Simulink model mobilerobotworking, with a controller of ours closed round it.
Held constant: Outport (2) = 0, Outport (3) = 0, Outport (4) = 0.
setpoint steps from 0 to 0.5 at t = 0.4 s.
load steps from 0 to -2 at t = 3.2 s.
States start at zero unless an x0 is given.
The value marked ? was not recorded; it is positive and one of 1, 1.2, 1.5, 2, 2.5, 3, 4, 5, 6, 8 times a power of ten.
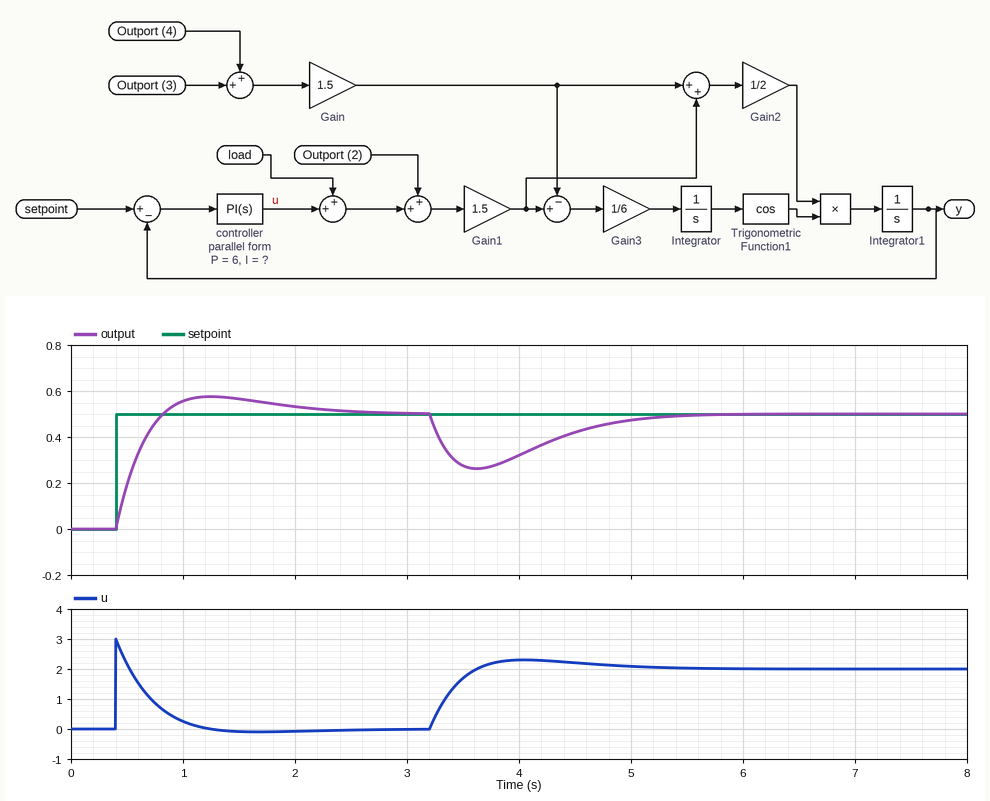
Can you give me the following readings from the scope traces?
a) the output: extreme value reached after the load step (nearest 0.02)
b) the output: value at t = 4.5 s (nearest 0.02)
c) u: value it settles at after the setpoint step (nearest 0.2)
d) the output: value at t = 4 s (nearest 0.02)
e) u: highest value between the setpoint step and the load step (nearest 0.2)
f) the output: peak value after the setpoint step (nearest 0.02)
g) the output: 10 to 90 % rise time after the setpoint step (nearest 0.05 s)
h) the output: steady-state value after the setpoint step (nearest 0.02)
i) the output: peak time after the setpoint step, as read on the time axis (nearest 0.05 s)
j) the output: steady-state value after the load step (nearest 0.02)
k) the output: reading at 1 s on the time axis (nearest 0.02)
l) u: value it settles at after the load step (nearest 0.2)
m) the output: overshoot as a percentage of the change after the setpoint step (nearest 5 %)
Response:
0.26
0.42
0.0
0.32
3.0
0.58
0.30 s
0.50
1.25 s
0.50
0.56
2.0
15 %
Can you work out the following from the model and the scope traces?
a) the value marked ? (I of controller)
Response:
8
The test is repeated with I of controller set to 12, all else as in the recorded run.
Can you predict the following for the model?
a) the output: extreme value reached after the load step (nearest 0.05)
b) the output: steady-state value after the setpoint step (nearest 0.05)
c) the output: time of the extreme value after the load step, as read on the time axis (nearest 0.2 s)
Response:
0.30
0.50
3.6 s
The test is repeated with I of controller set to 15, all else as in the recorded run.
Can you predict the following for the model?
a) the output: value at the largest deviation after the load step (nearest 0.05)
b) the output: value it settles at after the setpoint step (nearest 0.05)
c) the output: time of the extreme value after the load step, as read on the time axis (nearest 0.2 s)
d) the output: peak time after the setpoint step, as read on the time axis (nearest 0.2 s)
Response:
0.30
0.50
3.6 s
1.0 s
